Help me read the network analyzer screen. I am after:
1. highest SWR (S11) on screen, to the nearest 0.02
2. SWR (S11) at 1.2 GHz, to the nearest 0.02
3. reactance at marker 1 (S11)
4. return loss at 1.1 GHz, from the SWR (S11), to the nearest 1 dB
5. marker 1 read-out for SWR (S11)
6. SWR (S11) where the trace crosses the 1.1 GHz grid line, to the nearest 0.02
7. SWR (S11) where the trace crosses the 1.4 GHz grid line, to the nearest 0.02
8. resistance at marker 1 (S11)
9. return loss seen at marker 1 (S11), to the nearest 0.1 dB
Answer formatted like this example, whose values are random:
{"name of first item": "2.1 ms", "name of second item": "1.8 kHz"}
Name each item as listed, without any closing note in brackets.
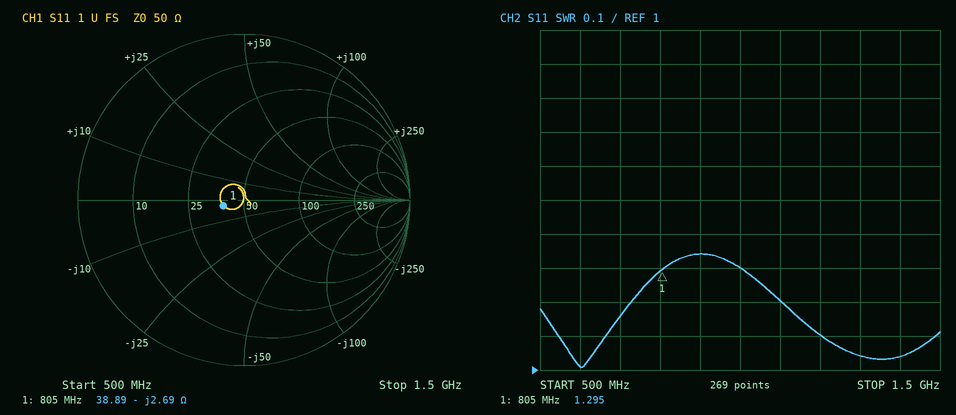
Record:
{"highest SWR (S11) on screen, to the nearest 0.02": "1.34", "SWR (S11) at 1.2 GHz, to the nearest 0.02": "1.10", "reactance at marker 1": "-2.69 Ω", "return loss at 1.1 GHz, from the SWR (S11), to the nearest 1 dB": "21 dB", "marker 1 read-out for SWR": "1.295", "SWR (S11) where the trace crosses the 1.1 GHz grid line, to the nearest 0.02": "1.20", "SWR (S11) where the trace crosses the 1.4 GHz grid line, to the nearest 0.02": "1.04", "resistance at marker 1": "38.89 Ω", "return loss seen at marker 1 (S11), to the nearest 0.1 dB": "17.8 dB"}
